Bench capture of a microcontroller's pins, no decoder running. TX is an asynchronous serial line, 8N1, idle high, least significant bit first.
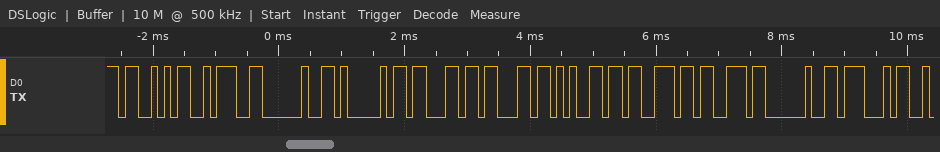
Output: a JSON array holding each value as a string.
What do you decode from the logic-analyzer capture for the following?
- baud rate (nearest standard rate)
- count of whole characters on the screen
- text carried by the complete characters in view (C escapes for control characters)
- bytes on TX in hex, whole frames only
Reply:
["9600 baud", "11", "\"S: Access G\"", "53 3A 20 41 63 63 65 73 73 20 47"]
